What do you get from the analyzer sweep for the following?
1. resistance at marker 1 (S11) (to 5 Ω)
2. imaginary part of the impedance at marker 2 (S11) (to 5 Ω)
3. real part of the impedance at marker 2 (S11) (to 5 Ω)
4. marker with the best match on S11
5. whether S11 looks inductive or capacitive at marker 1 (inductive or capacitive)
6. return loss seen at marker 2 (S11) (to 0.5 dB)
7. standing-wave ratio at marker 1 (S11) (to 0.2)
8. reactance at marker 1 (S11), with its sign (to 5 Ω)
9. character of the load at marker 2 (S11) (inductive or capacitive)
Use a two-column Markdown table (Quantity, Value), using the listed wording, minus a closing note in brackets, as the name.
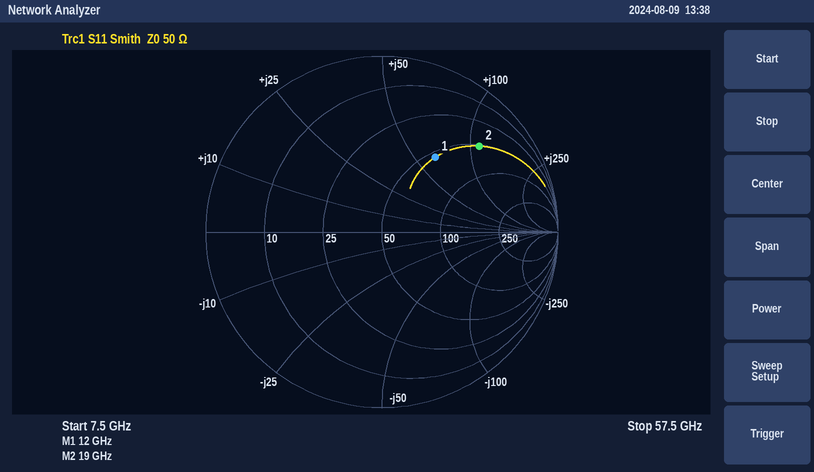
| Quantity | Value |
|---|---|
| resistance at marker 1 (S11) | 55 Ω |
| imaginary part of the impedance at marker 2 (S11) | +110 Ω |
| real part of the impedance at marker 2 (S11) | 50 Ω |
| marker with the best match on S11 | marker 1 |
| whether S11 looks inductive or capacitive at marker 1 | inductive |
| return loss seen at marker 2 (S11) | 2.5 dB |
| standing-wave ratio at marker 1 (S11) | 3.2 |
| reactance at marker 1 (S11), with its sign | +65 Ω |
| character of the load at marker 2 (S11) | inductive |
